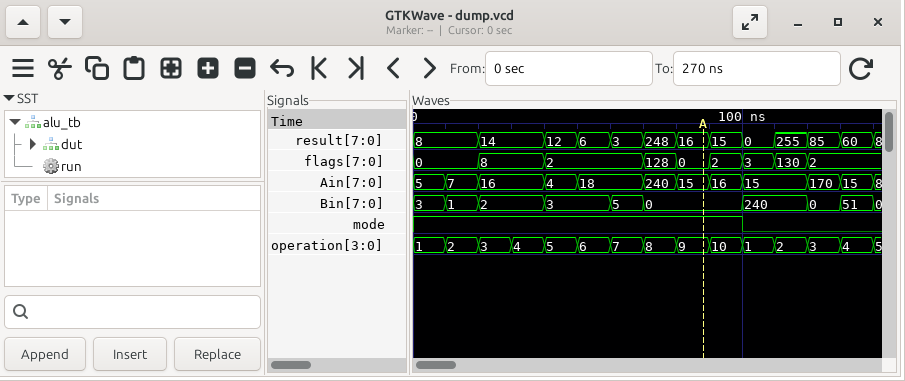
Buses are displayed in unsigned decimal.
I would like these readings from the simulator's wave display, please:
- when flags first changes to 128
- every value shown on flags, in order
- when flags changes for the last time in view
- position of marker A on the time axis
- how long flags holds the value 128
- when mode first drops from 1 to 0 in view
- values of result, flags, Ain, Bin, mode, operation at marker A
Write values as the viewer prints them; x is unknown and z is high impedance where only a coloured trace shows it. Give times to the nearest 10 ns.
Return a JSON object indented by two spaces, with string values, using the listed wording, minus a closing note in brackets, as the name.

{
  "when flags first changes to 128": "70 ns",
  "every value shown on flags, in order": "0, 8, 2, 128, 0, 2, 3, 130, 2",
  "when flags changes for the last time in view": "120 ns",
  "position of marker A on the time axis": "90 ns",
  "how long flags holds the value 128": "10 ns",
  "when mode first drops from 1 to 0 in view": "100 ns",
  "values of result, flags, Ain, Bin, mode, operation at marker A": "result=16, flags=0, Ain=15, Bin=0, mode=1, operation=9"
}
